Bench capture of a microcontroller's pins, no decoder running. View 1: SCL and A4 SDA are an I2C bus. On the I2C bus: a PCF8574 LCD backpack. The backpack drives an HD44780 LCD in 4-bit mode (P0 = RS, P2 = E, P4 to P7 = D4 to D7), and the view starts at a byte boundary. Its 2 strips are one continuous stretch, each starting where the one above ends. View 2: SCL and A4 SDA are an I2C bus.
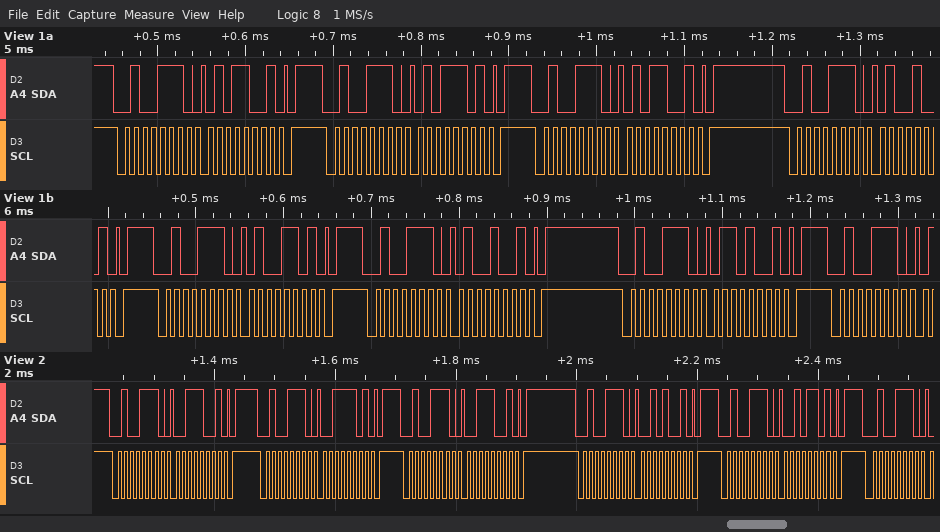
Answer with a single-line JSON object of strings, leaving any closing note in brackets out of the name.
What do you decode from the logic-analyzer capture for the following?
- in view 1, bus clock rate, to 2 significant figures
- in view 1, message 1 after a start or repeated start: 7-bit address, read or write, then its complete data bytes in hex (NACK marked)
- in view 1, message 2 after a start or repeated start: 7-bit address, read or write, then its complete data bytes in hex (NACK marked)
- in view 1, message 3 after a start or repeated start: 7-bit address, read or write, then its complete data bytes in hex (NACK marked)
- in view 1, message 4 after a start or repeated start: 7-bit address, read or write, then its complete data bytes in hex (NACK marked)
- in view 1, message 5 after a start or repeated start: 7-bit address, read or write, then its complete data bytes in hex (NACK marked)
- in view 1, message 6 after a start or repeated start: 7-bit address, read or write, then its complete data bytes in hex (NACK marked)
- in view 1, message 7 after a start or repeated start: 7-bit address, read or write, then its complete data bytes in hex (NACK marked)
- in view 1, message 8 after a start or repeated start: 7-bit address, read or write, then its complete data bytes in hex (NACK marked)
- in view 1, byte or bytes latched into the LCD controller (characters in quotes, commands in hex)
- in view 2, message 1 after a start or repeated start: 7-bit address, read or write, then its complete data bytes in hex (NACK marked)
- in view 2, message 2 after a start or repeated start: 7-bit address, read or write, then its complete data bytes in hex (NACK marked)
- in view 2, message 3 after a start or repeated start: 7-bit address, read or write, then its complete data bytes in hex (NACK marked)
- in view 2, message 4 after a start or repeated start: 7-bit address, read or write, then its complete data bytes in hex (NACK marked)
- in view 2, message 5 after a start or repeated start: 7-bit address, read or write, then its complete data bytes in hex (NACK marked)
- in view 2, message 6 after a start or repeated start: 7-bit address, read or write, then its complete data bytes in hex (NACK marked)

{"in view 1, bus clock rate, to 2 significant figures": "100 kHz", "in view 1, message 1 after a start or repeated start: 7-bit address, read or write, then its complete data bytes in hex": "0x27 write: 59", "in view 1, message 2 after a start or repeated start: 7-bit address, read or write, then its complete data bytes in hex": "0x27 write: 5D", "in view 1, message 3 after a start or repeated start: 7-bit address, read or write, then its complete data bytes in hex": "0x27 write: 59", "in view 1, message 4 after a start or repeated start: 7-bit address, read or write, then its complete data bytes in hex": "0x27 write: 49", "in view 1, message 5 after a start or repeated start: 7-bit address, read or write, then its complete data bytes in hex": "0x27 write: 4D", "in view 1, message 6 after a start or repeated start: 7-bit address, read or write, then its complete data bytes in hex": "0x27 write: 49", "in view 1, message 7 after a start or repeated start: 7-bit address, read or write, then its complete data bytes in hex": "0x27 write: 69", "in view 1, message 8 after a start or repeated start: 7-bit address, read or write, then its complete data bytes in hex": "0x27 write", "in view 1, byte or bytes latched into the LCD controller": "'T'", "in view 2, message 1 after a start or repeated start: 7-bit address, read or write, then its complete data bytes in hex": "0x27 write: 39", "in view 2, message 2 after a start or repeated start: 7-bit address, read or write, then its complete data bytes in hex": "0x27 write: 3D", "in view 2, message 3 after a start or repeated start: 7-bit address, read or write, then its complete data bytes in hex": "0x27 write: 39", "in view 2, message 4 after a start or repeated start: 7-bit address, read or write, then its complete data bytes in hex": "0x27 write: 29", "in view 2, message 5 after a start or repeated start: 7-bit address, read or write, then its complete data bytes in hex": "0x27 write: 2D", "in view 2, message 6 after a start or repeated start: 7-bit address, read or write, then its complete data bytes in hex": "0x27 write"}
